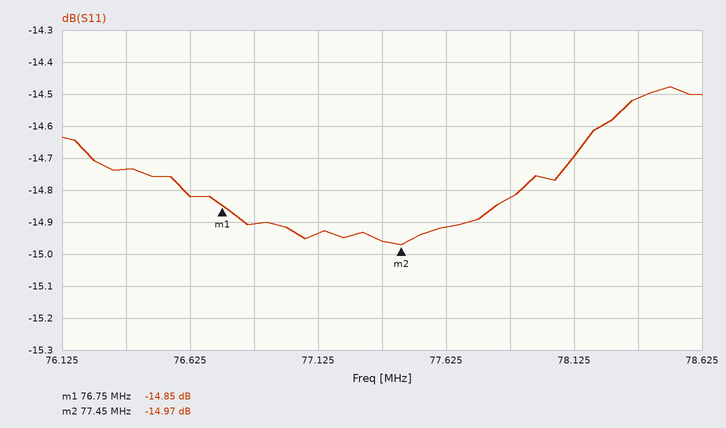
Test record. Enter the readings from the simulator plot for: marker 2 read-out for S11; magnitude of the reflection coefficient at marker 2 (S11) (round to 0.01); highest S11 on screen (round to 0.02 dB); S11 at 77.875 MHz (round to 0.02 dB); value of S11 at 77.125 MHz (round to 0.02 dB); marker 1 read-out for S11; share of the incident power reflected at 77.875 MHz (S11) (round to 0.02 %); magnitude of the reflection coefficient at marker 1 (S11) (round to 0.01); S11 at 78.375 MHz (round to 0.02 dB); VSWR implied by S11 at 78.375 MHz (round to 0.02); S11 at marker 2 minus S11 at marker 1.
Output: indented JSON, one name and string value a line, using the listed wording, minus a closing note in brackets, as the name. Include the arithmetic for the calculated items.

{
  "marker 2 read-out for S11": "-14.97 dB",
  "magnitude of the reflection coefficient at marker 2 (S11)": "10^(-14.97/20) ≈ 0.18",
  "highest S11 on screen": "-14.48 dB",
  "S11 at 77.875 MHz": "-14.82 dB",
  "value of S11 at 77.125 MHz": "-14.94 dB",
  "marker 1 read-out for S11": "-14.85 dB",
  "share of the incident power reflected at 77.875 MHz (S11)": "10^(-14.82/10) ≈ 3.30 %",
  "magnitude of the reflection coefficient at marker 1 (S11)": "10^(-14.85/20) ≈ 0.18",
  "S11 at 78.375 MHz": "-14.52 dB",
  "VSWR implied by S11 at 78.375 MHz": "|Γ| = 10^(-14.52/20) = 0.1879; VSWR = (1 + 0.1879)/(1 − 0.1879) ≈ 1.46",
  "S11 at marker 2 minus S11 at marker 1": "-14.97 − (-14.85) = -0.12 dB"
}
